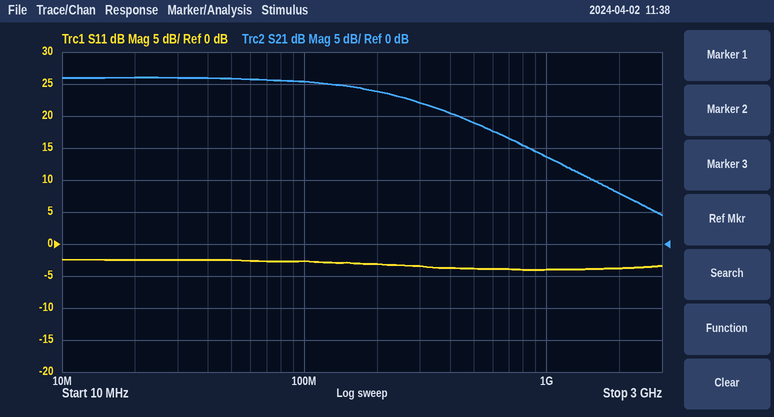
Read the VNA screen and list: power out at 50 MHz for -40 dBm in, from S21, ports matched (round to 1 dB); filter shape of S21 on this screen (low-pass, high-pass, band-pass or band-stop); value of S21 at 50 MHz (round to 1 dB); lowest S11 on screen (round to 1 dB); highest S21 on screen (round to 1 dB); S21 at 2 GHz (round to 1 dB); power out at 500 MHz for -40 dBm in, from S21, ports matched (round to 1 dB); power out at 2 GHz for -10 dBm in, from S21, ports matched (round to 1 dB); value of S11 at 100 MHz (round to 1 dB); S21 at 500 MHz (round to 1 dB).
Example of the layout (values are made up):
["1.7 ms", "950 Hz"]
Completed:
["-14 dBm", "low-pass", "26 dB", "-4 dB", "26 dB", "8 dB", "-21 dBm", "-2 dBm", "-3 dB", "19 dB"]
